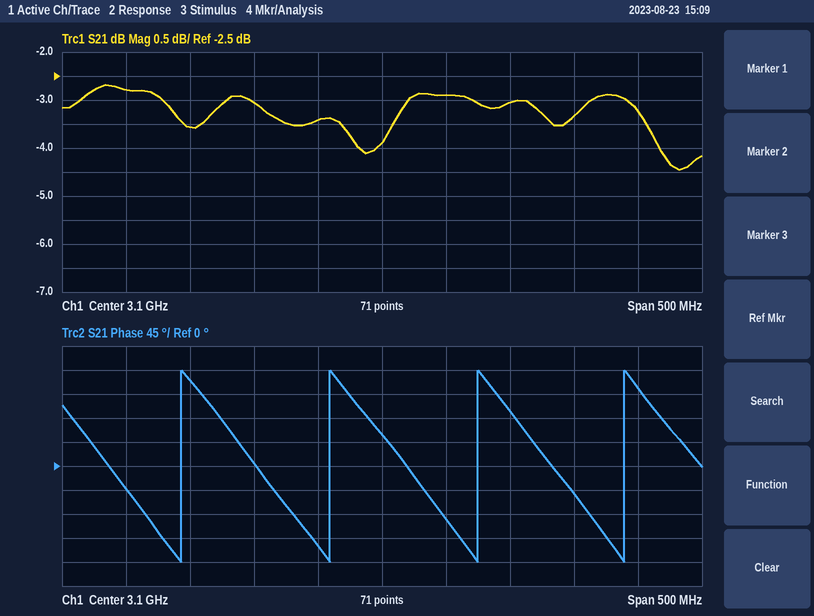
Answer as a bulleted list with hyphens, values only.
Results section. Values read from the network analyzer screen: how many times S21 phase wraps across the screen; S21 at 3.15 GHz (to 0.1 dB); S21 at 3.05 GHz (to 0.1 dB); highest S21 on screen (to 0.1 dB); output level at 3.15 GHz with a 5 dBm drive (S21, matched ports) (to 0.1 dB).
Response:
- 4
- -2.9 dB
- -3.4 dB
- -2.7 dB
- 2.1 dBm
